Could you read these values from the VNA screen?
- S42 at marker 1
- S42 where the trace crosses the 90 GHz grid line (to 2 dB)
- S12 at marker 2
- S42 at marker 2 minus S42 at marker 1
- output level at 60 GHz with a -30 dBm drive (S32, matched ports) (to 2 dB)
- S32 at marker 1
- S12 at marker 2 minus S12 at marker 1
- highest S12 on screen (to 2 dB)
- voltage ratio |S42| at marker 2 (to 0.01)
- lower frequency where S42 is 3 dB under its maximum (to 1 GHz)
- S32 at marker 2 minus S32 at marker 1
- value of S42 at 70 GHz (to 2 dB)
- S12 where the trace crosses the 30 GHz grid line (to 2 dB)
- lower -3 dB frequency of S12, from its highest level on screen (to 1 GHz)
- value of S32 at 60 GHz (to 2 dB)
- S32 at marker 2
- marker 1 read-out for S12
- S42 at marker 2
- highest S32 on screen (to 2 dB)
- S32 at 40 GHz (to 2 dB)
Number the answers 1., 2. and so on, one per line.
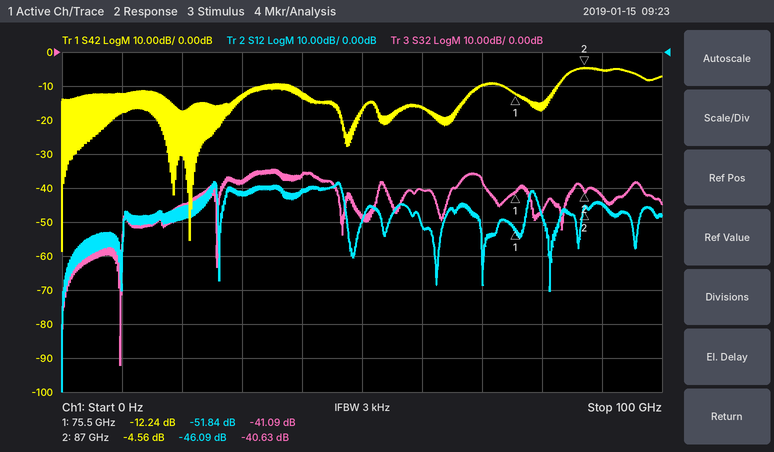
1. -12.24 dB
2. -6 dB
3. -46.09 dB
4. 7.68 dB
5. -70 dBm
6. -41.09 dB
7. 5.75 dB
8. -38 dB
9. 0.59
10. 84 GHz
11. 0.46 dB
12. -10 dB
13. -42 dB
14. 25 GHz
15. -40 dB
16. -40.63 dB
17. -51.84 dB
18. -4.56 dB
19. -34 dB
20. -36 dB
